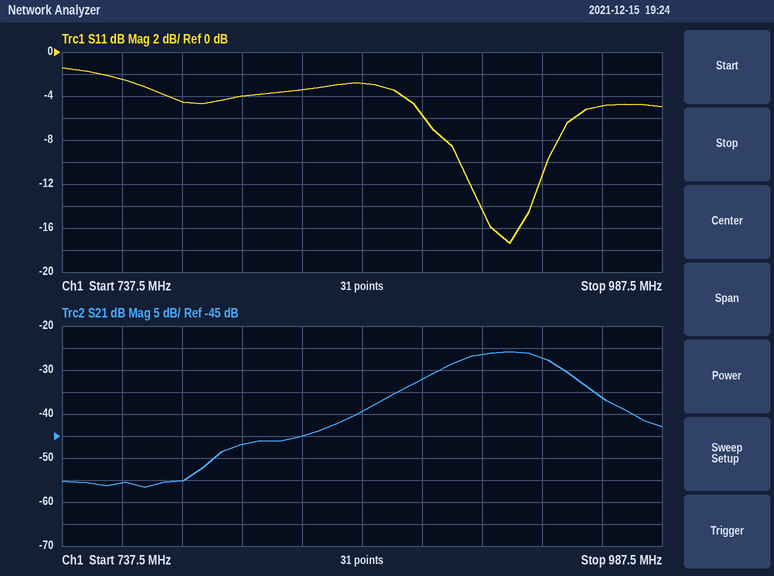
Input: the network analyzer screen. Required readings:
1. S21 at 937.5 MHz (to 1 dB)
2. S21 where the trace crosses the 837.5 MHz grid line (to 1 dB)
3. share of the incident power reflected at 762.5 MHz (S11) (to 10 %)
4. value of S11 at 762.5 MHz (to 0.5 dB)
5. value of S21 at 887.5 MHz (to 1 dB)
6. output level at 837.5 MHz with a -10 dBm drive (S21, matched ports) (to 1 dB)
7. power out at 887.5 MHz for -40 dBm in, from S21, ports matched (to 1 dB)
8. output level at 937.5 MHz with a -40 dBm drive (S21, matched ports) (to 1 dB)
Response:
-27 dB
-45 dB
60 %
-2.5 dB
-32 dB
-55 dBm
-72 dBm
-67 dBm
